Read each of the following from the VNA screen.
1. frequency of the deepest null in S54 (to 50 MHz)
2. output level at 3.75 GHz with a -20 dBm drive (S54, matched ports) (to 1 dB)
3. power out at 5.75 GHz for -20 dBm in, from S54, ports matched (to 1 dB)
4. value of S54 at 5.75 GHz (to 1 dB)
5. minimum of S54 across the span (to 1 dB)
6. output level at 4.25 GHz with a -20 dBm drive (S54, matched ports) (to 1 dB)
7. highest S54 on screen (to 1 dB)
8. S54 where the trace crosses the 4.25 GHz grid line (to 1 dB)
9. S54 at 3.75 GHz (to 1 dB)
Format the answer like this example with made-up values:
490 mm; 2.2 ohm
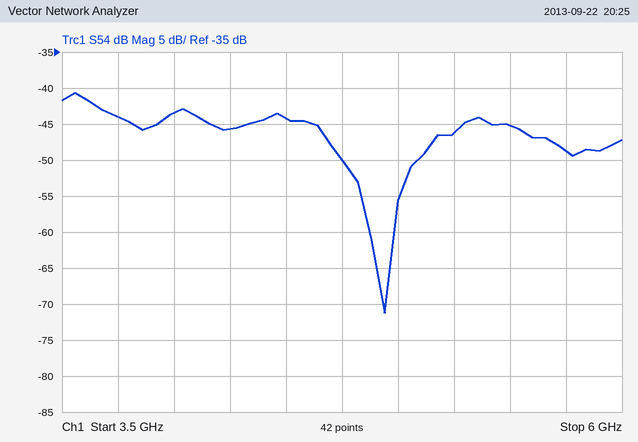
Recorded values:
4.95 GHz; -64 dBm; -69 dBm; -49 dB; -71 dB; -66 dBm; -41 dB; -46 dB; -44 dB
